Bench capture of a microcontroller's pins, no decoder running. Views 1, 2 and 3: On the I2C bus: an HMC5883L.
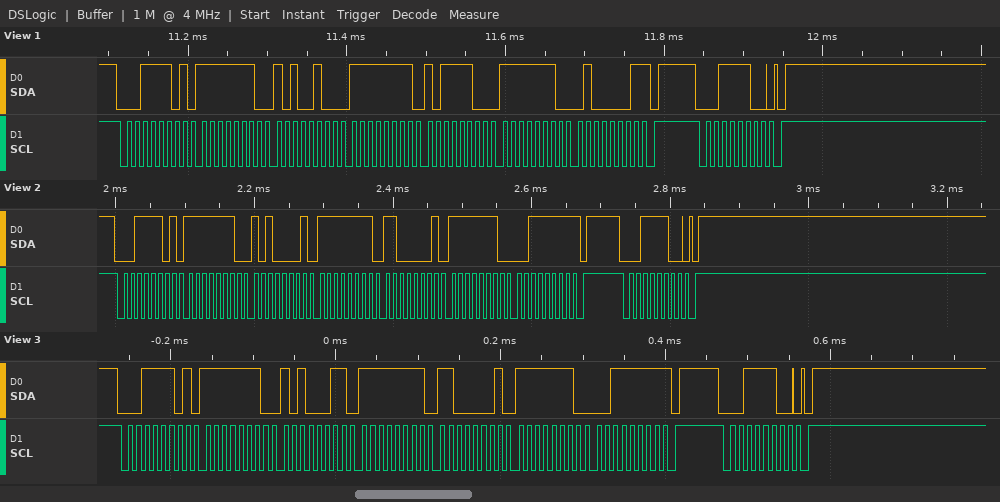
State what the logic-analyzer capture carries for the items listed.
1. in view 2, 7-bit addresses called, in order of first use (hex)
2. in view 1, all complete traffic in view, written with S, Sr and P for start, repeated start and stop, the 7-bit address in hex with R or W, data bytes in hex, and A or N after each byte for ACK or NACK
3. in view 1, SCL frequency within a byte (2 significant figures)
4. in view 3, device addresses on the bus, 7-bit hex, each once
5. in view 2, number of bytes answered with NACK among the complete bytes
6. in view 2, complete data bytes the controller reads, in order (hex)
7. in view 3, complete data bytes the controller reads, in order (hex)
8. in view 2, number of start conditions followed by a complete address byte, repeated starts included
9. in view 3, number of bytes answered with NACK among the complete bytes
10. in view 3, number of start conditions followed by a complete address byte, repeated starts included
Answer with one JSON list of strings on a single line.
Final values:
["0x1E", "S 1ER A FE A A4 A FF A BC A FE A 41 N P S 1EW A P", "100 kHz", "0x1E", "1", "FE A1 FF C1 FE 3F", "FE A3 FF C1 FE 3F", "2", "1", "2"]
